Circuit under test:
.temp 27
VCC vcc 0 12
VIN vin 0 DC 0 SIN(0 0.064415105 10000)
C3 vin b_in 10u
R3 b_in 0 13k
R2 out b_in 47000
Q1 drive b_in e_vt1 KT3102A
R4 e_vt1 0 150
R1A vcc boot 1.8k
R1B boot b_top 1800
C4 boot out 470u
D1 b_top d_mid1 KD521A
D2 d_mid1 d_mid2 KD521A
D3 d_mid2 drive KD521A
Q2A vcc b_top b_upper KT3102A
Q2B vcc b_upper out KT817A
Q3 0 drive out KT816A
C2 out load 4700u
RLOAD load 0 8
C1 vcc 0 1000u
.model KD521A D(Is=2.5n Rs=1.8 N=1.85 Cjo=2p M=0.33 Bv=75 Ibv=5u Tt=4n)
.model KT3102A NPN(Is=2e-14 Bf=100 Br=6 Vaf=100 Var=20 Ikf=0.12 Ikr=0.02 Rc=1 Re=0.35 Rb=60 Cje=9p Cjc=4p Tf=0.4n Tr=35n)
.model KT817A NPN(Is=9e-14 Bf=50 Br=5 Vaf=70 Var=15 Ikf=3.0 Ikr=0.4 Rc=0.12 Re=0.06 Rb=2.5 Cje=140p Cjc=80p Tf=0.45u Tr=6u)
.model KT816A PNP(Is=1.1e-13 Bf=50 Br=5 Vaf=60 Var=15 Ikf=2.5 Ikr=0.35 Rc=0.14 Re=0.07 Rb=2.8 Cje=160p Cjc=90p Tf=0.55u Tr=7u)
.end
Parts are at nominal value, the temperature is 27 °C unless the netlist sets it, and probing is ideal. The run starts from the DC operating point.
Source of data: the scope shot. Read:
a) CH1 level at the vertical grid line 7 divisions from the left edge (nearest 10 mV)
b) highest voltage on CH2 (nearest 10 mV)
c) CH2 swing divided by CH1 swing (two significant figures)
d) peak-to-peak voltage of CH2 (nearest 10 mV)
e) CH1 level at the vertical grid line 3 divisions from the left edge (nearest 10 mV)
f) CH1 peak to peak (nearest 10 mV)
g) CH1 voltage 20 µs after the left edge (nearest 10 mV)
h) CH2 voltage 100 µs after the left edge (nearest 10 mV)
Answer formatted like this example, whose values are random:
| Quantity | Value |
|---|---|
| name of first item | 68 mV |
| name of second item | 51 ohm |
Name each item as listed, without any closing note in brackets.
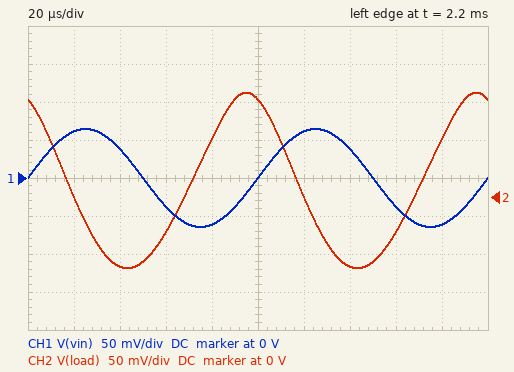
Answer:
| Quantity | Value |
|---|---|
| CH1 level at the vertical grid line 7 divisions from the left edge | 40 mV |
| highest voltage on CH2 | 140 mV |
| CH2 swing divided by CH1 swing | 1.8 |
| peak-to-peak voltage of CH2 | 230 mV |
| CH1 level at the vertical grid line 3 divisions from the left edge | -40 mV |
| CH1 peak to peak | 130 mV |
| CH1 voltage 20 µs after the left edge | 60 mV |
| CH2 voltage 100 µs after the left edge | 130 mV |
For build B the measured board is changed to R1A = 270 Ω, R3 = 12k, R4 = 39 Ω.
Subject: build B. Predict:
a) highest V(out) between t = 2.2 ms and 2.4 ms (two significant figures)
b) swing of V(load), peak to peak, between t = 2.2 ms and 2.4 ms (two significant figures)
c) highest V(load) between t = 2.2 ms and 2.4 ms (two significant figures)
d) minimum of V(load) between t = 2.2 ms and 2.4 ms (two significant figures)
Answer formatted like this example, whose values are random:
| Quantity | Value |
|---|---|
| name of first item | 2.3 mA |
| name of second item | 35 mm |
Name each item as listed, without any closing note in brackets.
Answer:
| Quantity | Value |
|---|---|
| highest V(out) between t = 2.2 ms and 2.4 ms | 6.1 V |
| swing of V(load), peak to peak, between t = 2.2 ms and 2.4 ms | 1.0 V |
| highest V(load) between t = 2.2 ms and 2.4 ms | 720 mV |
| minimum of V(load) between t = 2.2 ms and 2.4 ms | -310 mV |
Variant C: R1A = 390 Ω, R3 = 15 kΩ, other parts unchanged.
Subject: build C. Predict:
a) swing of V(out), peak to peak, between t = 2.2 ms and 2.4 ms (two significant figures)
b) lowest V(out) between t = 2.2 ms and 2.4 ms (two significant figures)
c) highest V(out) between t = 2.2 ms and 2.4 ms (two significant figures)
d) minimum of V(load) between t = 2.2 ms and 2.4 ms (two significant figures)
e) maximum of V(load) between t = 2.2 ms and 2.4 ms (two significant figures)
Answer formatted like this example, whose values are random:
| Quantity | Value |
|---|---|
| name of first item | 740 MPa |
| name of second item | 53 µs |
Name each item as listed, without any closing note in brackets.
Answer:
| Quantity | Value |
|---|---|
| swing of V(out), peak to peak, between t = 2.2 ms and 2.4 ms | 220 mV |
| lowest V(out) between t = 2.2 ms and 2.4 ms | 5.7 V |
| highest V(out) between t = 2.2 ms and 2.4 ms | 5.9 V |
| minimum of V(load) between t = 2.2 ms and 2.4 ms | -100 mV |
| maximum of V(load) between t = 2.2 ms and 2.4 ms | 120 mV |
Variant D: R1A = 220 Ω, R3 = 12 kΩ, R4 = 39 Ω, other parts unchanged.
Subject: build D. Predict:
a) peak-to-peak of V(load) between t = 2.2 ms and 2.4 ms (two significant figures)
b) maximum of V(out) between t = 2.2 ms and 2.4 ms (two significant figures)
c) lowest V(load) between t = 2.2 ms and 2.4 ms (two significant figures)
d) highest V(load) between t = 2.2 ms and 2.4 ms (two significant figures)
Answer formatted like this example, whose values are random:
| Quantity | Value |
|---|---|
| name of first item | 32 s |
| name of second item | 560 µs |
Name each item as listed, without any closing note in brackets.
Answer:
| Quantity | Value |
|---|---|
| peak-to-peak of V(load) between t = 2.2 ms and 2.4 ms | 970 mV |
| maximum of V(out) between t = 2.2 ms and 2.4 ms | 6.1 V |
| lowest V(load) between t = 2.2 ms and 2.4 ms | -310 mV |
| highest V(load) between t = 2.2 ms and 2.4 ms | 660 mV |
